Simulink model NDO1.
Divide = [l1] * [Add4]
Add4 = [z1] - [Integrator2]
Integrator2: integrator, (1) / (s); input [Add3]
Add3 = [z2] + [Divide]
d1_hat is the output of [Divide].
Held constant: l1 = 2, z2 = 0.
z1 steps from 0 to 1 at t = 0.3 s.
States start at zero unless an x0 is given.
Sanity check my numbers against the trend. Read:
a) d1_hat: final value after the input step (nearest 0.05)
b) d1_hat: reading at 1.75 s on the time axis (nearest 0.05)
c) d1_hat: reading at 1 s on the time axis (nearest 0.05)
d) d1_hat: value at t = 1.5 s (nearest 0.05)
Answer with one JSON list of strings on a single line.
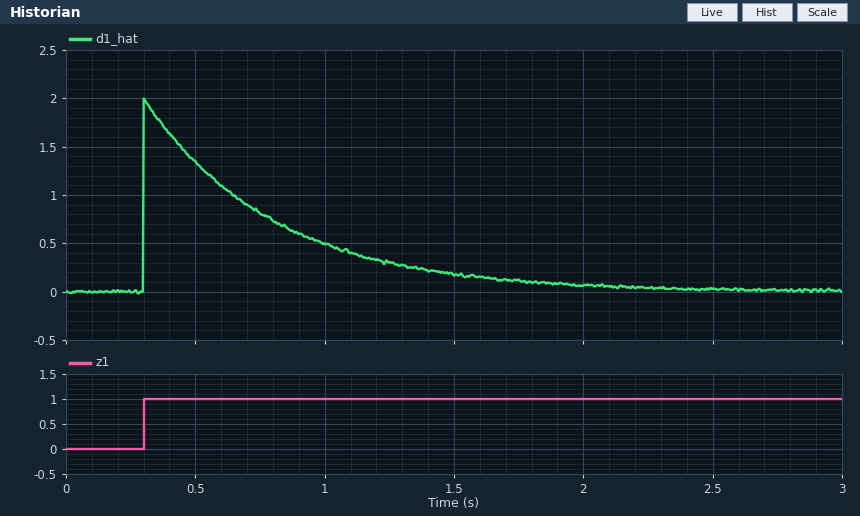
["0.00", "0.10", "0.50", "0.20"]
